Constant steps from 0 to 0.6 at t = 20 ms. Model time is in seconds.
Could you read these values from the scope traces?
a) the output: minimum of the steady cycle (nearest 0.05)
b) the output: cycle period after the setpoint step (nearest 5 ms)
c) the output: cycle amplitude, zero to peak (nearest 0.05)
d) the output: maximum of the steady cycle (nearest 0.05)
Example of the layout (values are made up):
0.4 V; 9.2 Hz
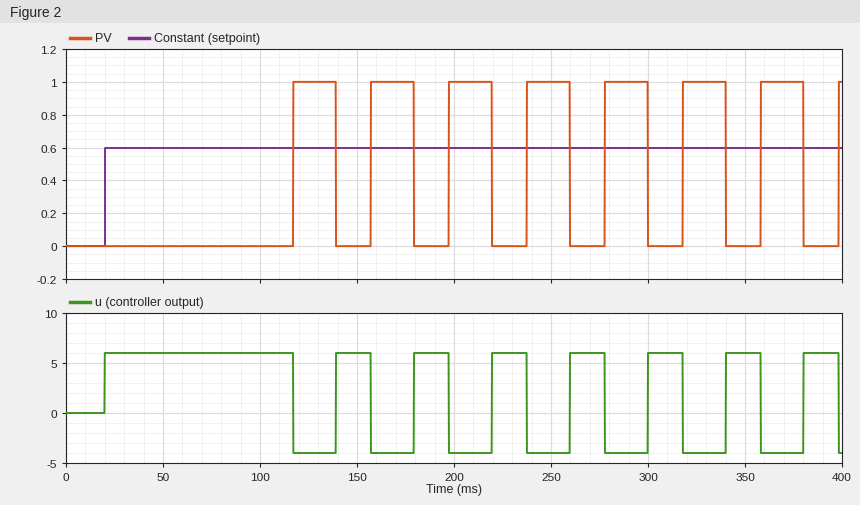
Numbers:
0.00; 40 ms; 0.50; 1.00
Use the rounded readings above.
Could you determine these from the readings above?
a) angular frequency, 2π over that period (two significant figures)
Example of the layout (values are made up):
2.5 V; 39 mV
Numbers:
0.16 rad/ms
